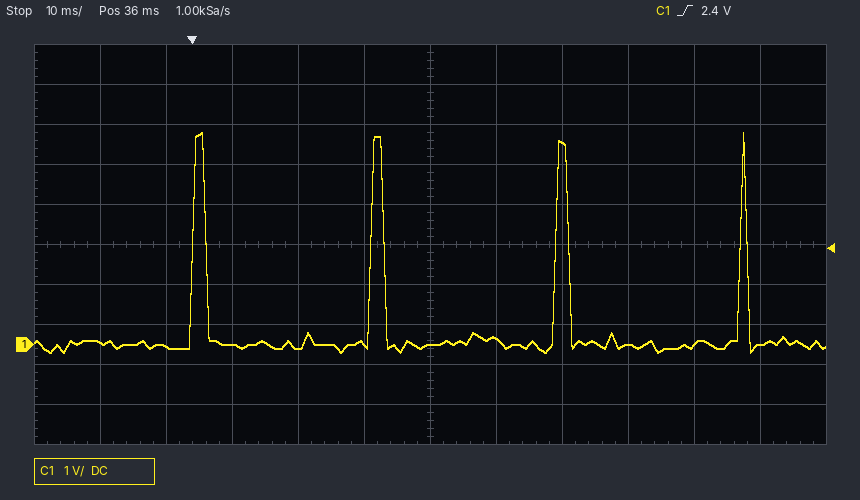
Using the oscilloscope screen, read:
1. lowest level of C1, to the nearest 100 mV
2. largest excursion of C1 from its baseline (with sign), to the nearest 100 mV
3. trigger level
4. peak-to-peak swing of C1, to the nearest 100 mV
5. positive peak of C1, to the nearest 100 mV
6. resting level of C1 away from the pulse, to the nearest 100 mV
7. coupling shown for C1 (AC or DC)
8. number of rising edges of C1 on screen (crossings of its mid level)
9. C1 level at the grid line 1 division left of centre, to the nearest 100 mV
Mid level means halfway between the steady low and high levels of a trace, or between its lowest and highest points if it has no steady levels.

-200 mV
+5.3 V
2.4 V
5.5 V
5.3 V
0.0 V
DC
4
0.0 V
